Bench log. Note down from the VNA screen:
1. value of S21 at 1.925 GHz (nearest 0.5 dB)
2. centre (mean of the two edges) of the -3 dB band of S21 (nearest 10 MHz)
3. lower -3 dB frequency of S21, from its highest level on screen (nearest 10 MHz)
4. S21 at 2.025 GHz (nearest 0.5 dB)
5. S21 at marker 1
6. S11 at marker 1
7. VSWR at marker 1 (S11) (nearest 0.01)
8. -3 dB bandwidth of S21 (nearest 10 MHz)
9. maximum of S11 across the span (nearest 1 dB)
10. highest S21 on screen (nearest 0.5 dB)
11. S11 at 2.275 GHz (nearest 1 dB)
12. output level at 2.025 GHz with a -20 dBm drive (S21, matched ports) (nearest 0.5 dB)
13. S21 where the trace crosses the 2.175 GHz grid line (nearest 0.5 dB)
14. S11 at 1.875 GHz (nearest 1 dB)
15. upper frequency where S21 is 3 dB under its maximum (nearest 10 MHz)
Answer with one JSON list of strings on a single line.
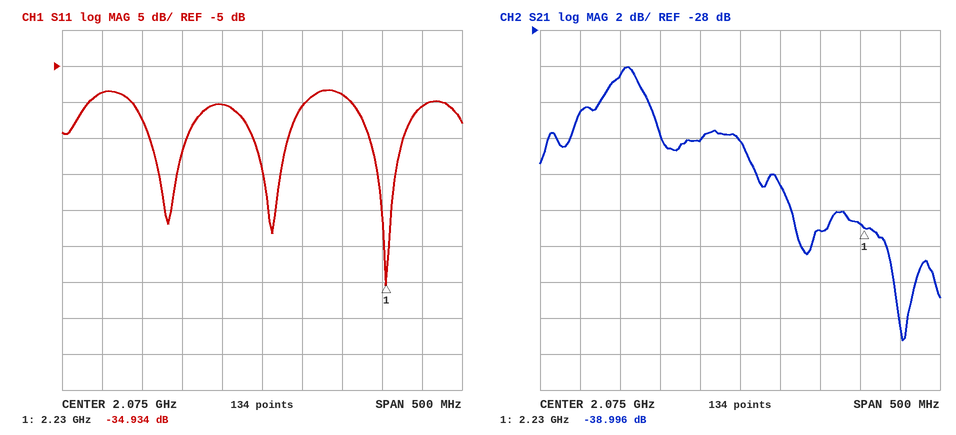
["-30.5 dB", "1.92 GHz", "1.87 GHz", "-34.0 dB", "-38.996 dB", "-34.934 dB", "1.04", "100 MHz", "-8 dB", "-30.0 dB", "-11 dB", "-54.0 dBm", "-39.0 dB", "-9 dB", "1.97 GHz"]
